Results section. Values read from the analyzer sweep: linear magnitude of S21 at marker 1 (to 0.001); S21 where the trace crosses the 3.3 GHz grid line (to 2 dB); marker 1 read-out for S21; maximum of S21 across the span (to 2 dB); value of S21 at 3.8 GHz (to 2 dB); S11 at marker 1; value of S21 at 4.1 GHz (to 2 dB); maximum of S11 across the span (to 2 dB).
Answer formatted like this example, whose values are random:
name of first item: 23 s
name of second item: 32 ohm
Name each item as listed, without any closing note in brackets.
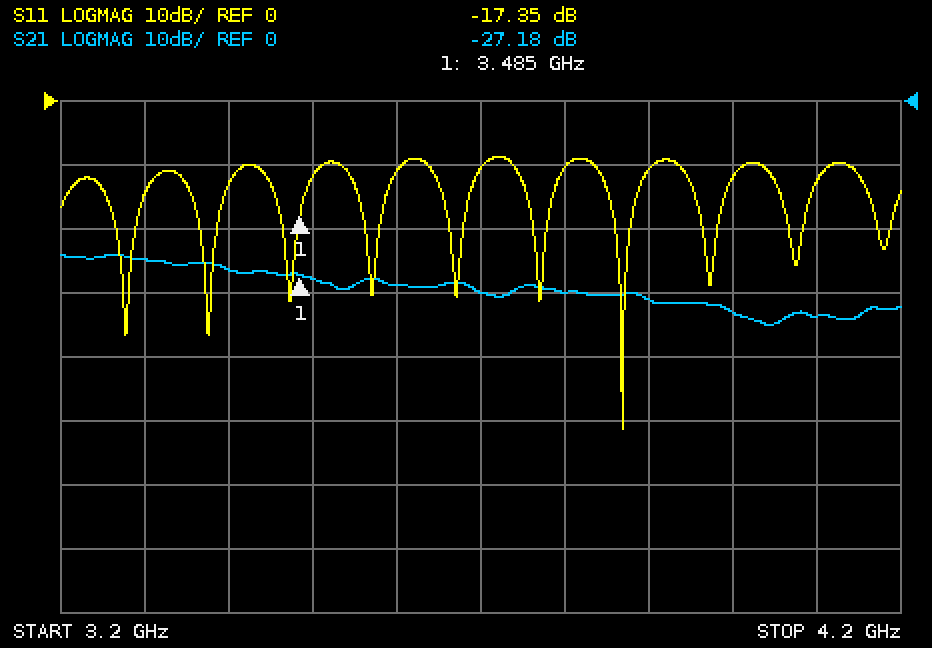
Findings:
linear magnitude of S21 at marker 1: 0.044
S21 where the trace crosses the 3.3 GHz grid line: -24 dB
marker 1 read-out for S21: -27.18 dB
maximum of S21 across the span: -24 dB
value of S21 at 3.8 GHz: -30 dB
S11 at marker 1: -17.35 dB
value of S21 at 4.1 GHz: -34 dB
maximum of S11 across the span: -8 dB
